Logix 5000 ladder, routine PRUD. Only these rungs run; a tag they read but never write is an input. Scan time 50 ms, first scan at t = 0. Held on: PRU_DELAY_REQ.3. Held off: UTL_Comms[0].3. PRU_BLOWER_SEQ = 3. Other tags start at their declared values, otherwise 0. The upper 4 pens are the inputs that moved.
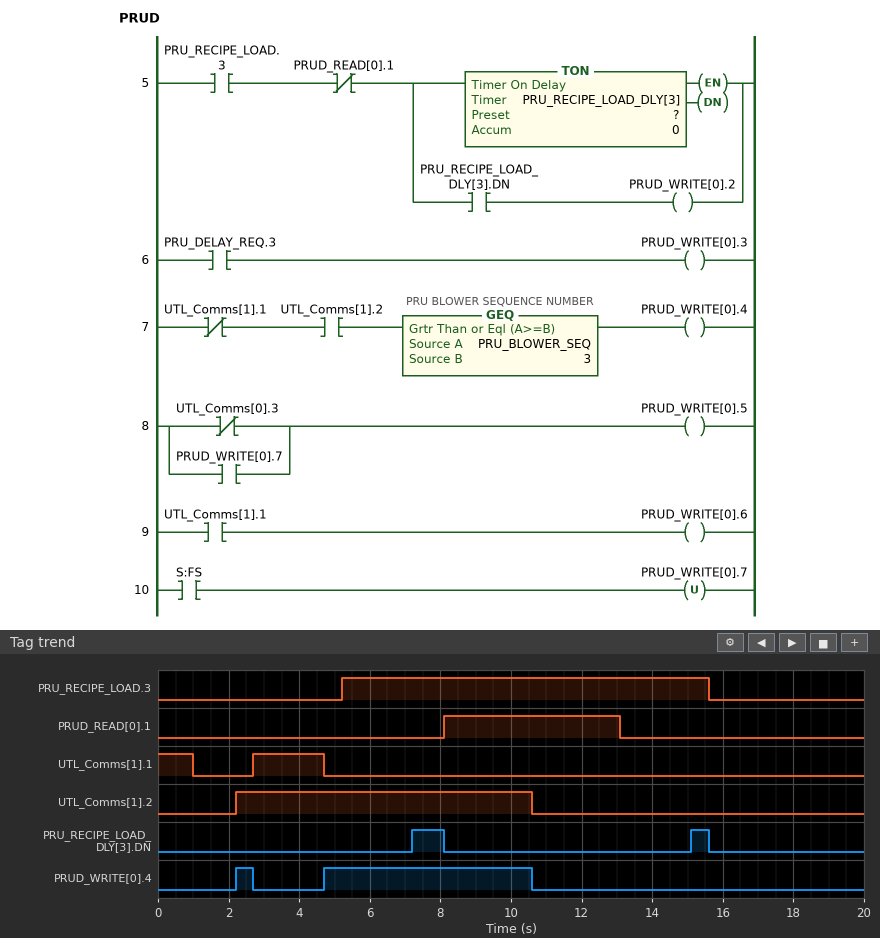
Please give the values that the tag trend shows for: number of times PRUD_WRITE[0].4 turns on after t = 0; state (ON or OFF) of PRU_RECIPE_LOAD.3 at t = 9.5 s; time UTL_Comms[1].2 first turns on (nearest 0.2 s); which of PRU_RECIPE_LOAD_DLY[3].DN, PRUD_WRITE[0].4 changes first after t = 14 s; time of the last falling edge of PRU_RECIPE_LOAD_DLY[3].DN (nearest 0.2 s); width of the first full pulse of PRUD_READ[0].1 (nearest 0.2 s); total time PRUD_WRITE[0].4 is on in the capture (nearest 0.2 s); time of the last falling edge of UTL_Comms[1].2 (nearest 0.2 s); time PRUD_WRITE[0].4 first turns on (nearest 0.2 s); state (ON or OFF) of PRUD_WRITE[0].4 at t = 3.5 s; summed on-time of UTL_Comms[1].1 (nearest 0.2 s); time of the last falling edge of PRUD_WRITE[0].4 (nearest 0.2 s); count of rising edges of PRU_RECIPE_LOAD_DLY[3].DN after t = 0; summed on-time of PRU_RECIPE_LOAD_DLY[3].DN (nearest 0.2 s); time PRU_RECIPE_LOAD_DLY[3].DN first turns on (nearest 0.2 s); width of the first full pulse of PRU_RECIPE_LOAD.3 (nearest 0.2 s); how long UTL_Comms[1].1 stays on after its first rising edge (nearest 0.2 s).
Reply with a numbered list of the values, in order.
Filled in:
1. 2
2. ON
3. 2.2 s
4. PRU_RECIPE_LOAD_DLY[3].DN
5. 15.6 s
6. 5.0 s
7. 6.4 s
8. 10.6 s
9. 2.2 s
10. OFF
11. 3.0 s
12. 10.6 s
13. 2
14. 1.4 s
15. 7.2 s
16. 10.4 s
17. 2.0 s
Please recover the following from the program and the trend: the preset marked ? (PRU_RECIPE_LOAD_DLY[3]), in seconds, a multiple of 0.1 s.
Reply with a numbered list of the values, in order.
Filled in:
1. 2.0 s
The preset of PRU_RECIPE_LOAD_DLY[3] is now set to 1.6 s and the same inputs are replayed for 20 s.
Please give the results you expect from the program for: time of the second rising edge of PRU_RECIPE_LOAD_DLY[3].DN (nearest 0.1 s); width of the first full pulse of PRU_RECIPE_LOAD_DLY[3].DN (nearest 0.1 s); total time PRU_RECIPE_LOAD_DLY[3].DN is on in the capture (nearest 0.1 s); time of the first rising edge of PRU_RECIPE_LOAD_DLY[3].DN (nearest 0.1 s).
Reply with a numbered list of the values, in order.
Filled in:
1. 14.7 s
2. 1.3 s
3. 2.2 s
4. 6.8 s
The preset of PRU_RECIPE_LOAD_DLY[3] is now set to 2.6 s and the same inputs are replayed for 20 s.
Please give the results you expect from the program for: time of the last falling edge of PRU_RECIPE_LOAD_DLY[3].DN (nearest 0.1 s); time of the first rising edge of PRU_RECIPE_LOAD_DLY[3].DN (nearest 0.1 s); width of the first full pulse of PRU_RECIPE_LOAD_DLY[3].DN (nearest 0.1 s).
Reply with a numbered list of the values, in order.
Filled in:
1. 8.1 s
2. 7.8 s
3. 0.3 s
